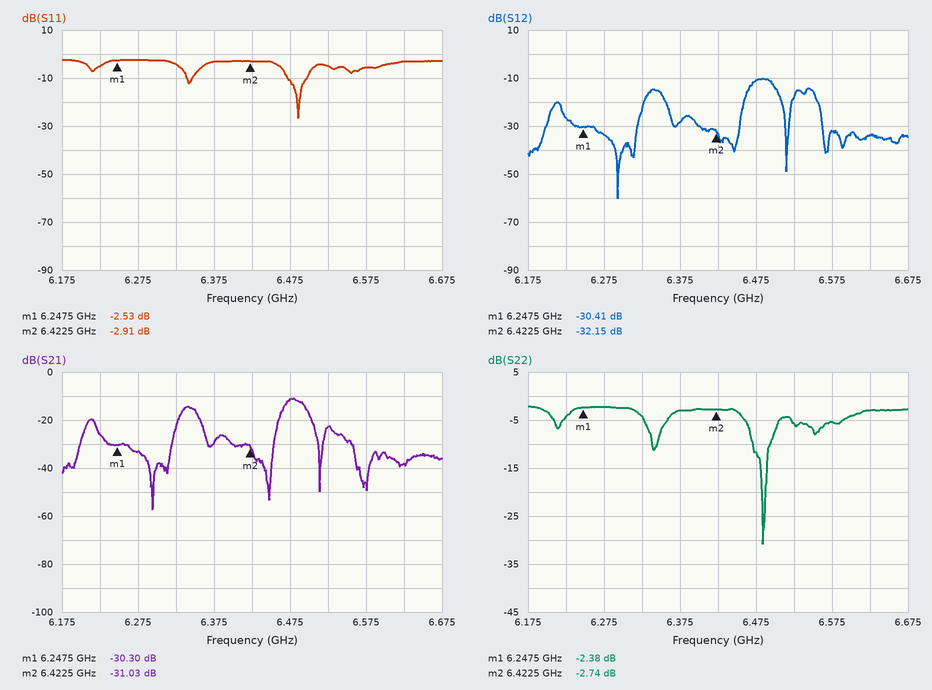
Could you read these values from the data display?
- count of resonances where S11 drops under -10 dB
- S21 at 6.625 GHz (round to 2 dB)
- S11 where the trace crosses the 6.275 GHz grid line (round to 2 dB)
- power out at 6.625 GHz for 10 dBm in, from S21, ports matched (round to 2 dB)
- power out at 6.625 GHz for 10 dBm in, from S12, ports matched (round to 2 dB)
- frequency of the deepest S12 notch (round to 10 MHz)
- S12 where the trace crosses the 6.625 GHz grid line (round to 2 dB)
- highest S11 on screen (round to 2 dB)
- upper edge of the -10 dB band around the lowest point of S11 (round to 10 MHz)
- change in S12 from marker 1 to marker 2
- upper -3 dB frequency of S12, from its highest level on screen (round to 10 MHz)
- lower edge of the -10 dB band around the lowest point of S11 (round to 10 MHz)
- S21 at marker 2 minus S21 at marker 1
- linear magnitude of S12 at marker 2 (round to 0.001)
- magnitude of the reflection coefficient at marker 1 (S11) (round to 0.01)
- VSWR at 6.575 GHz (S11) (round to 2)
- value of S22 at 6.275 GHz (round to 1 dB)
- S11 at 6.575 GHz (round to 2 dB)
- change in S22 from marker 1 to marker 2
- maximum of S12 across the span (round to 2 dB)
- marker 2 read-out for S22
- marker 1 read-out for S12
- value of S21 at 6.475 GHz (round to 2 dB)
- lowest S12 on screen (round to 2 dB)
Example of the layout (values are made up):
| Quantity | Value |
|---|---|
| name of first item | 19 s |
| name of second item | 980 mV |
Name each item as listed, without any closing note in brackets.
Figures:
| Quantity | Value |
|---|---|
| count of resonances where S11 drops under -10 dB | 2 |
| S21 at 6.625 GHz | -38 dB |
| S11 where the trace crosses the 6.275 GHz grid line | -2 dB |
| power out at 6.625 GHz for 10 dBm in, from S21, ports matched | -28 dBm |
| power out at 6.625 GHz for 10 dBm in, from S12, ports matched | -24 dBm |
| frequency of the deepest S12 notch | 6.29 GHz |
| S12 where the trace crosses the 6.625 GHz grid line | -34 dB |
| highest S11 on screen | -2 dB |
| upper edge of the -10 dB band around the lowest point of S11 | 6.50 GHz |
| change in S12 from marker 1 to marker 2 | -1.74 dB |
| upper -3 dB frequency of S12, from its highest level on screen | 6.50 GHz |
| lower edge of the -10 dB band around the lowest point of S11 | 6.47 GHz |
| S21 at marker 2 minus S21 at marker 1 | -0.73 dB |
| linear magnitude of S12 at marker 2 | 0.025 |
| magnitude of the reflection coefficient at marker 1 (S11) | 0.75 |
| VSWR at 6.575 GHz (S11) | 4 |
| value of S22 at 6.275 GHz | -2 dB |
| S11 at 6.575 GHz | -6 dB |
| change in S22 from marker 1 to marker 2 | -0.36 dB |
| maximum of S12 across the span | -10 dB |
| marker 2 read-out for S22 | -2.74 dB |
| marker 1 read-out for S12 | -30.41 dB |
| value of S21 at 6.475 GHz | -12 dB |
| lowest S12 on screen | -60 dB |
